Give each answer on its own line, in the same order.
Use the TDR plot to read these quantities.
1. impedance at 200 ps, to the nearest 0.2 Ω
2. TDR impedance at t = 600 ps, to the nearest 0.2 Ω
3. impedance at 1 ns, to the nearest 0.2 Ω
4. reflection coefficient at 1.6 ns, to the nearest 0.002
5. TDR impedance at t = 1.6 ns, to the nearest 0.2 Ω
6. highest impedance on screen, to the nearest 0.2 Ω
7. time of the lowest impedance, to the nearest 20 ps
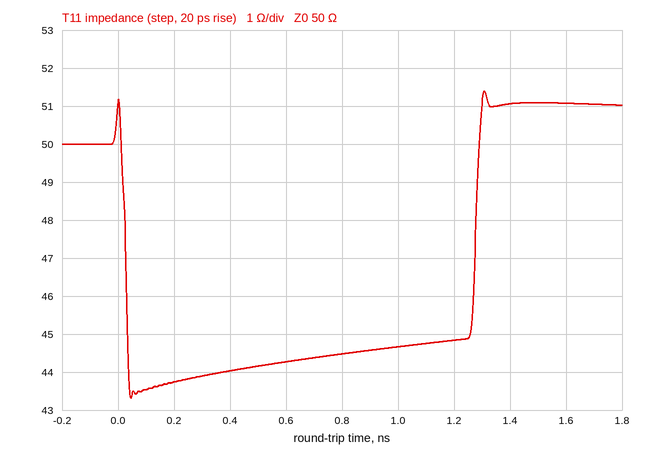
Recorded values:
43.8 Ω
44.2 Ω
44.6 Ω
+0.010
51.0 Ω
51.4 Ω
40 ps
